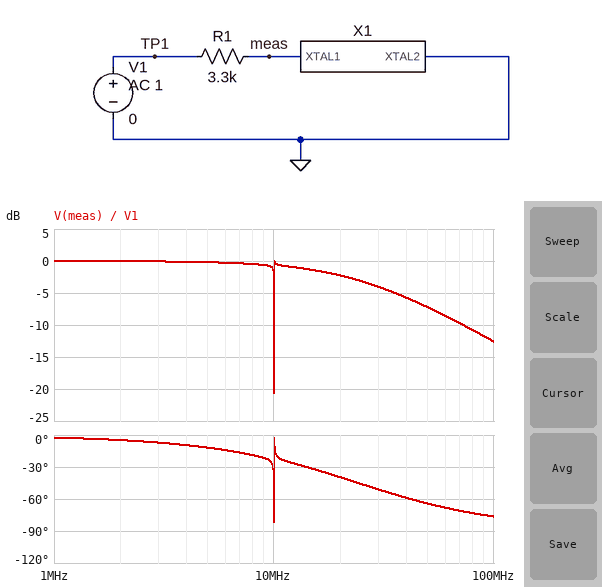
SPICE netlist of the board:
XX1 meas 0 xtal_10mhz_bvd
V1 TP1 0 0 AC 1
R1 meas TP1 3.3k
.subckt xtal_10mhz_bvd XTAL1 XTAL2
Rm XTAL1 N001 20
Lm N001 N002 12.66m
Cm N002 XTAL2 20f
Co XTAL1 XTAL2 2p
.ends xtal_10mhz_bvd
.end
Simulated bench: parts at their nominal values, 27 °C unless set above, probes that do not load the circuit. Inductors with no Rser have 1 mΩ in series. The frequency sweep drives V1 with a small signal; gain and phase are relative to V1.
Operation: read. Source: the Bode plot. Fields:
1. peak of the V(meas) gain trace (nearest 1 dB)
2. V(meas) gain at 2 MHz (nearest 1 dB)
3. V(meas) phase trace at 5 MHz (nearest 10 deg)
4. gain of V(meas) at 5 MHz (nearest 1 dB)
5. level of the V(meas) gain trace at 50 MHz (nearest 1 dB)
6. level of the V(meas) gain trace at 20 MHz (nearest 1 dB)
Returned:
0 dB
0 dB
-10 deg
0 dB
-7 dB
-2 dB
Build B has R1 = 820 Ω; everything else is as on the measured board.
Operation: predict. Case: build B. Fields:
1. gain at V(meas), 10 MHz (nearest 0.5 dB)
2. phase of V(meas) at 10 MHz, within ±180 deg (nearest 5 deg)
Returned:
-9.0 dB
-65 deg
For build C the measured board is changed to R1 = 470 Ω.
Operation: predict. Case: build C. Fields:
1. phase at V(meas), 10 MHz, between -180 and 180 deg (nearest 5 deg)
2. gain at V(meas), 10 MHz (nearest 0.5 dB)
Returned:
-55 deg
-5.5 dB
